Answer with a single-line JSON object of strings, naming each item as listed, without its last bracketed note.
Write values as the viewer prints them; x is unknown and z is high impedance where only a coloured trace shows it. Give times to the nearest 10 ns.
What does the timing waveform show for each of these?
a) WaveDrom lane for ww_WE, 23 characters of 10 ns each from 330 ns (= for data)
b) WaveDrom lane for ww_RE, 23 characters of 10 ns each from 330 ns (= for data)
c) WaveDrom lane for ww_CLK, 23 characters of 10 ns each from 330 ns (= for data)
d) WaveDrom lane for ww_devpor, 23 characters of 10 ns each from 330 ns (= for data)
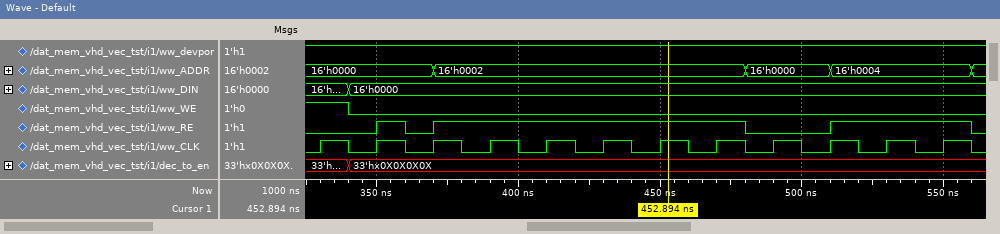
{"WaveDrom lane for ww_WE, 23 characters of 10 ns each from 330 ns": "{name: 'ww_WE', wave: '10.....................'}", "WaveDrom lane for ww_RE, 23 characters of 10 ns each from 330 ns": "{name: 'ww_RE', wave: '0.101..........0..1....'}", "WaveDrom lane for ww_CLK, 23 characters of 10 ns each from 330 ns": "{name: 'ww_CLK', wave: '10101010101010101010101'}", "WaveDrom lane for ww_devpor, 23 characters of 10 ns each from 330 ns": "{name: 'ww_devpor', wave: '1......................'}"}
